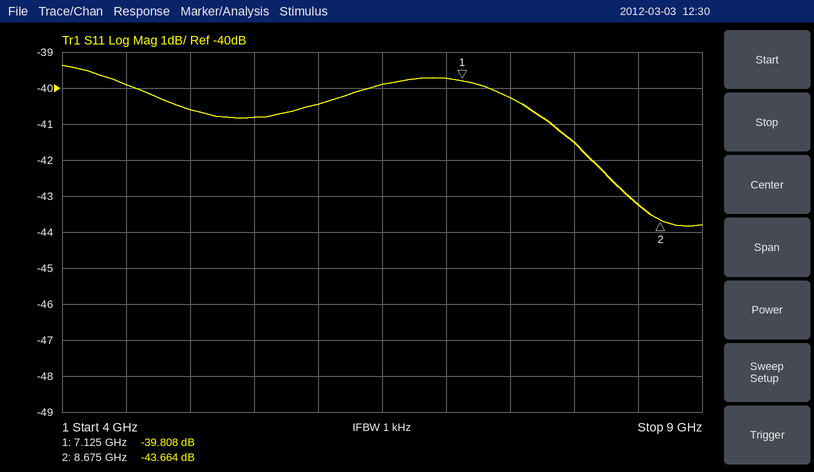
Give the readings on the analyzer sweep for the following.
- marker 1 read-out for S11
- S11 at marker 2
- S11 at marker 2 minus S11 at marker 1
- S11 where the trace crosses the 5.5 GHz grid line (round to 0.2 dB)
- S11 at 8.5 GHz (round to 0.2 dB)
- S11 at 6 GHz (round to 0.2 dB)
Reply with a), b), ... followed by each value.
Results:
a) -39.808 dB
b) -43.664 dB
c) -3.856 dB
d) -40.8 dB
e) -43.2 dB
f) -40.4 dB
